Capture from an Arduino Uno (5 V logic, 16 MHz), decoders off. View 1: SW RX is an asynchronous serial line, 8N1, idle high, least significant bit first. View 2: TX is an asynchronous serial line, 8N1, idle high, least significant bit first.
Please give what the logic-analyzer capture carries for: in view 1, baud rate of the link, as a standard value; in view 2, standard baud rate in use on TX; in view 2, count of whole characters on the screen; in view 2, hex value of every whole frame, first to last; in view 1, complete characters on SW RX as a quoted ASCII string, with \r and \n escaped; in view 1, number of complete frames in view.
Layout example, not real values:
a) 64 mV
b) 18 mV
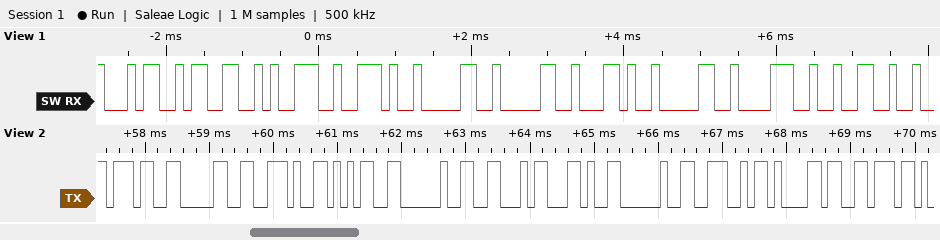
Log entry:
a) 9600 baud
b) 9600 baud
c) 11
d) 0x37 0x30 0x2E 0x35 0x20 0x46 0x2C 0x20 0x4E 0x61 0x76
e) "439.00,082"
f) 10
